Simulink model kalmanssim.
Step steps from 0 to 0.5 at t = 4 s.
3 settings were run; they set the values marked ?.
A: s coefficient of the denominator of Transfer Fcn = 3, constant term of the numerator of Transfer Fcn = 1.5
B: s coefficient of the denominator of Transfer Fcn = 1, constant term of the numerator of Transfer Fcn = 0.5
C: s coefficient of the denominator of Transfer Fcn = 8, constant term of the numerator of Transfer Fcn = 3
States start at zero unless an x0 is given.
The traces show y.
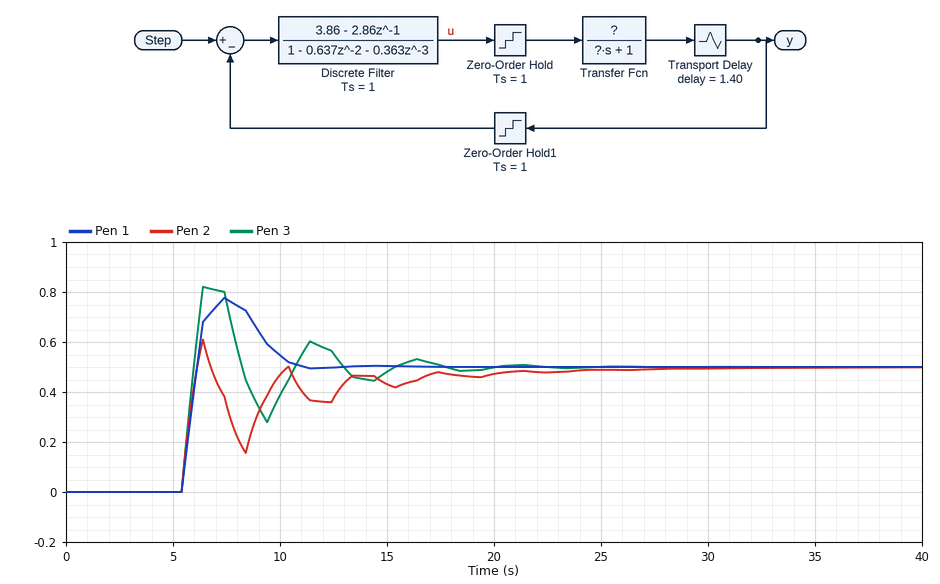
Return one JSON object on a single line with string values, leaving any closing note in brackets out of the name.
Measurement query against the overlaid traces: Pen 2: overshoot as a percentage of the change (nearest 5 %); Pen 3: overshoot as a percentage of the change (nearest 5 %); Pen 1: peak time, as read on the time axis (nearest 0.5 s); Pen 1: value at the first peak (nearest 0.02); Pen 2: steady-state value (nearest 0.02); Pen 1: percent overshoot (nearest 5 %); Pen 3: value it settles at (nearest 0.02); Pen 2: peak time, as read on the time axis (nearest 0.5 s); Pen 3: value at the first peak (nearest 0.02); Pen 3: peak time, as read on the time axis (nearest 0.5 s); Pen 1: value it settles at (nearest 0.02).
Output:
{"Pen 2: overshoot as a percentage of the change": "20 %", "Pen 3: overshoot as a percentage of the change": "65 %", "Pen 1: peak time, as read on the time axis": "7.5 s", "Pen 1: value at the first peak": "0.78", "Pen 2: steady-state value": "0.50", "Pen 1: percent overshoot": "55 %", "Pen 3: value it settles at": "0.50", "Pen 2: peak time, as read on the time axis": "6.5 s", "Pen 3: value at the first peak": "0.82", "Pen 3: peak time, as read on the time axis": "6.5 s", "Pen 1: value it settles at": "0.50"}
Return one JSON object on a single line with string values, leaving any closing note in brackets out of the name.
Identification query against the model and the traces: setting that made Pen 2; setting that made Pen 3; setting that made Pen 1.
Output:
{"setting that made Pen 2": "B", "setting that made Pen 3": "A", "setting that made Pen 1": "C"}
